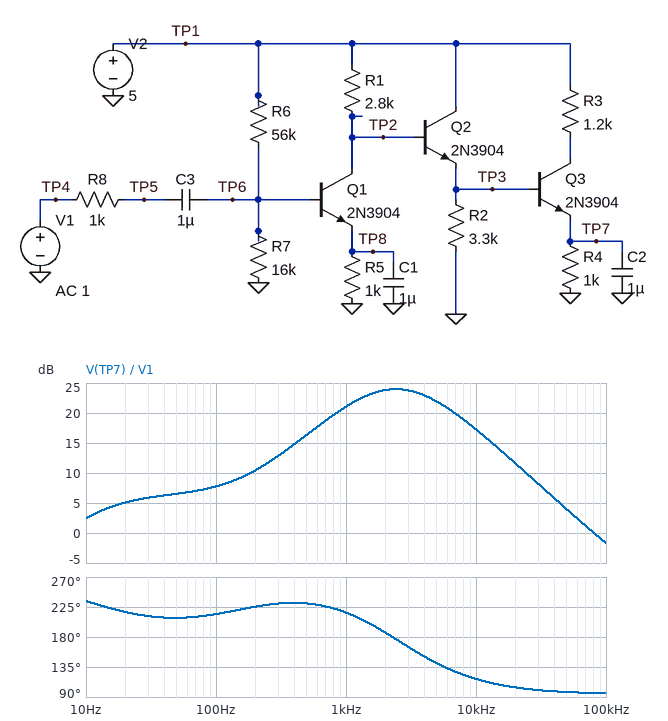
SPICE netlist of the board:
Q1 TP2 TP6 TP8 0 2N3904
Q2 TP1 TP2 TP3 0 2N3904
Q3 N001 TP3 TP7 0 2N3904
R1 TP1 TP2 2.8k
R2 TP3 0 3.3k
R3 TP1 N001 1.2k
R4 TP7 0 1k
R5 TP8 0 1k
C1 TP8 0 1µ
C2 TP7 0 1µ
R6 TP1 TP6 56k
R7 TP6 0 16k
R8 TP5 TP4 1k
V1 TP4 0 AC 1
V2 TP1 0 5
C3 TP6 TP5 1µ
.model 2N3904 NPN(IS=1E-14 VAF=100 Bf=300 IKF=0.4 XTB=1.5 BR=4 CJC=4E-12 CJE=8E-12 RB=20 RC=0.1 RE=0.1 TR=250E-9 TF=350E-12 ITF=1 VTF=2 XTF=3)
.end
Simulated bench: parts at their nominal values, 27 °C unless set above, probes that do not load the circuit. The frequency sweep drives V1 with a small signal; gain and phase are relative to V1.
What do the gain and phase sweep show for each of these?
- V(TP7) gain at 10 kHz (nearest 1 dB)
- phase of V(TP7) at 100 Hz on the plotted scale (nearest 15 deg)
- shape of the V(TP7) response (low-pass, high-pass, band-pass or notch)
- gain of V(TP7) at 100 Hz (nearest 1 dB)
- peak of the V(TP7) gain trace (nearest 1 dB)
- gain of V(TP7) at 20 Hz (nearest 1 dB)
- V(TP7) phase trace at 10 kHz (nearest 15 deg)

17 dB
210 deg
band-pass
8 dB
24 dB
5 dB
120 deg
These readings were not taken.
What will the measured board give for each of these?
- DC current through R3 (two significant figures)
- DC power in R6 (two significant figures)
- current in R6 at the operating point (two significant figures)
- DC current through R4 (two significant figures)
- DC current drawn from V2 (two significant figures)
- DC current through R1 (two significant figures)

2.2 mA
270 µW
70 µA
2.4 mA
3.8 mA
460 µA
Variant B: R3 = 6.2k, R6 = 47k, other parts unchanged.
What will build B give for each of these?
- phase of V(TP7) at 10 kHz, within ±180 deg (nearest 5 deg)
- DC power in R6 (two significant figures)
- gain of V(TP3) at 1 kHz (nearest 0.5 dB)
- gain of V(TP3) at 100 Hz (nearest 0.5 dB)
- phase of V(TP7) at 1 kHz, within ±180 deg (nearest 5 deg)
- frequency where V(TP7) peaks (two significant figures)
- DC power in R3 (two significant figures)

125 deg
300 µW
23.0 dB
9.0 dB
-135 deg
3.2 kHz
1.6 mW
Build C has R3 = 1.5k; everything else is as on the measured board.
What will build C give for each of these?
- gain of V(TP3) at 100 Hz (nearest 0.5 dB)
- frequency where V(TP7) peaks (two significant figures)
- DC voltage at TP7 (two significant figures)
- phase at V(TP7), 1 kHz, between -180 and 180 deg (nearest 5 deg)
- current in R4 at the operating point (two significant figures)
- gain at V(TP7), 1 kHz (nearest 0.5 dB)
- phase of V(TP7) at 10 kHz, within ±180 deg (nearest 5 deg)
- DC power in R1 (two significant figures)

8.5 dB
2.6 kHz
2.3 V
-140 deg
2.3 mA
21.5 dB
120 deg
600 µW
